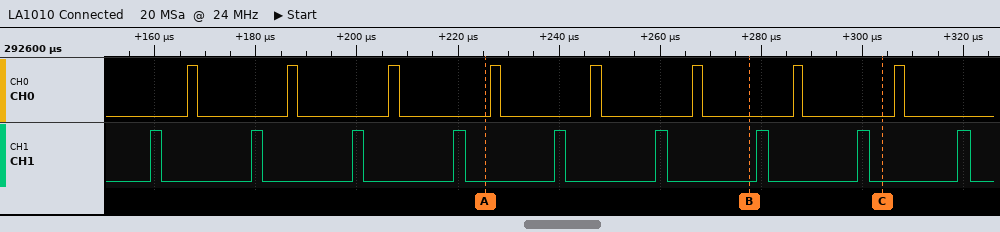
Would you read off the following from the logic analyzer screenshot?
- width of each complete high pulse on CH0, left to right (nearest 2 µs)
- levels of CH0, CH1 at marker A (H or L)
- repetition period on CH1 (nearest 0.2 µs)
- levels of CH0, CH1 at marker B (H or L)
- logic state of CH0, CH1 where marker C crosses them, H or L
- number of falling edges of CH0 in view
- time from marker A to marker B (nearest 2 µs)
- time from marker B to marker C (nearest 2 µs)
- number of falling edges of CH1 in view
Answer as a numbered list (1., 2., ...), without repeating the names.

1. 2 µs, 2 µs, 2 µs, 2 µs, 2 µs, 2 µs, 2 µs, 2 µs
2. CH0=L, CH1=L
3. 20 µs
4. CH0=L, CH1=L
5. CH0=L, CH1=L
6. 8
7. 52 µs
8. 26 µs
9. 9
